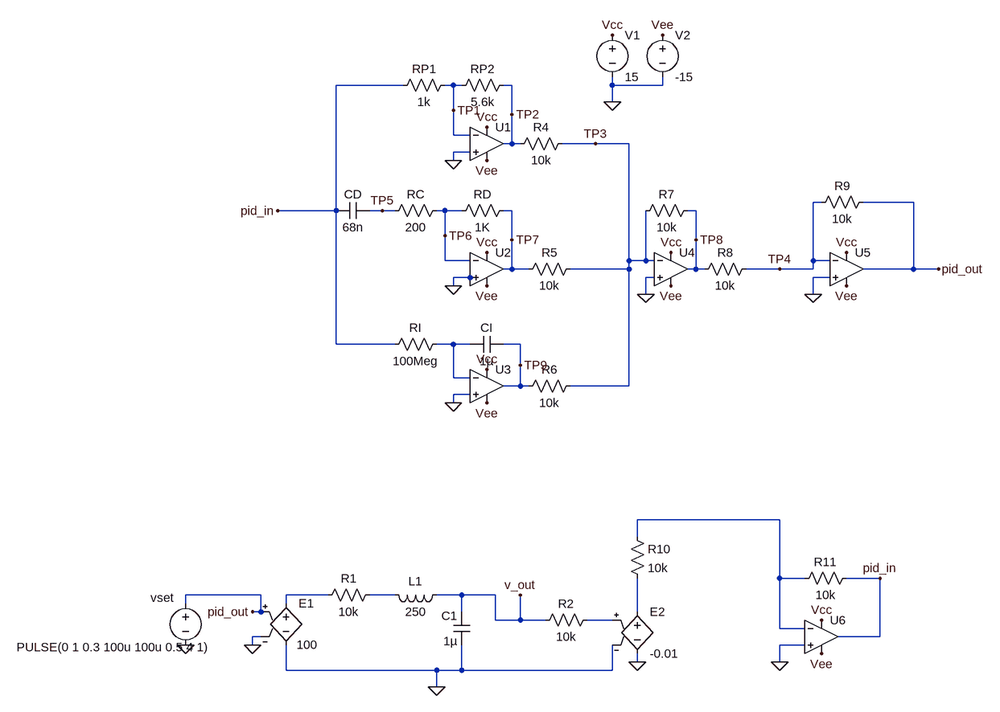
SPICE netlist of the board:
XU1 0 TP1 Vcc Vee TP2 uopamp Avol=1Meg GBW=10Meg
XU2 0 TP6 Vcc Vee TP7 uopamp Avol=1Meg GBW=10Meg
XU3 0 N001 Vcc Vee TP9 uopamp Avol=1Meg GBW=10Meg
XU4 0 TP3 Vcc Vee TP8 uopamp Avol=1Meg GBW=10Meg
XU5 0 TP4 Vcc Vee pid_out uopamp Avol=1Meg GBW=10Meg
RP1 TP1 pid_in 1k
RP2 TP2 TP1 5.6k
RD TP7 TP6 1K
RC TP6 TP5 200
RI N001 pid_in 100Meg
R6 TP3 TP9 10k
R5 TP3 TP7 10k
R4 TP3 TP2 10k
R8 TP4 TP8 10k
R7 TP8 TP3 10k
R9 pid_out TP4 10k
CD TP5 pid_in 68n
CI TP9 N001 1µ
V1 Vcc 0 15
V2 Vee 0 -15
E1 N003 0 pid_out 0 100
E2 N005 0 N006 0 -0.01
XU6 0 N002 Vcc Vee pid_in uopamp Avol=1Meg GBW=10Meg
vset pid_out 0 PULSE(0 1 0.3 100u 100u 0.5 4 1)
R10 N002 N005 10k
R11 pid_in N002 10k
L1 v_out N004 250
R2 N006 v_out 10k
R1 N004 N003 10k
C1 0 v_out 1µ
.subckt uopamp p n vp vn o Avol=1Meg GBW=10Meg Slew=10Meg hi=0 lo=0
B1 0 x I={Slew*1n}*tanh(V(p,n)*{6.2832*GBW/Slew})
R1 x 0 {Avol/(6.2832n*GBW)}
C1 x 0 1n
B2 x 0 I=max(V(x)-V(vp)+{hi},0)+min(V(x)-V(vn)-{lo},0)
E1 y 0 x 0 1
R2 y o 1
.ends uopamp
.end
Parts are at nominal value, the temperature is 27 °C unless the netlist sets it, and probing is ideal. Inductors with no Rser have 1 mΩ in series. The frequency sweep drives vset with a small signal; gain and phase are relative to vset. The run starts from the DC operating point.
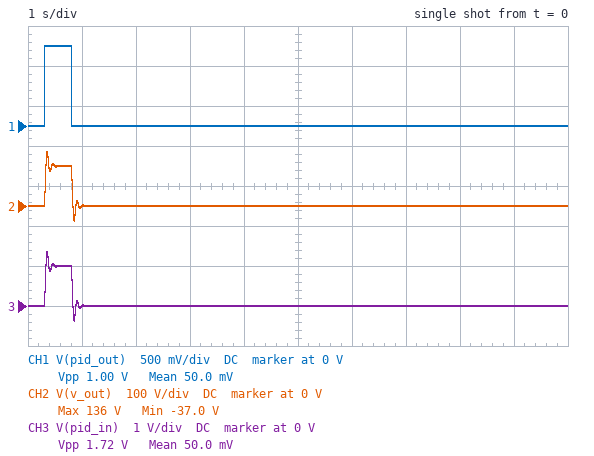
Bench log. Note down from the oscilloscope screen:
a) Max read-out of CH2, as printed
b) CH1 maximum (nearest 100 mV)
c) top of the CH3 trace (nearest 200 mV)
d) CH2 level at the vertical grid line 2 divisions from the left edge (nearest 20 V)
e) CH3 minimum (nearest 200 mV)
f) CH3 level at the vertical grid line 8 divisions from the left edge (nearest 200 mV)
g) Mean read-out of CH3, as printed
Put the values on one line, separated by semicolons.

136 V; 1.0 V; 1.4 V; 0 V; -400 mV; 0 V; 50.0 mV
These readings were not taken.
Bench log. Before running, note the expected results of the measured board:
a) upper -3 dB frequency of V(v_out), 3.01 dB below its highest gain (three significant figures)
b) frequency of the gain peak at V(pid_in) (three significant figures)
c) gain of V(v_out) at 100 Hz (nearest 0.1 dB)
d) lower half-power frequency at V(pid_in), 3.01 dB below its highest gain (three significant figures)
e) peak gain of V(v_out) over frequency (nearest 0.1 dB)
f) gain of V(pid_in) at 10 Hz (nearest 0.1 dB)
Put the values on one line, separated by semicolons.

11.9 Hz; 9.00 Hz; 0.2 dB; 4.50 Hz; 44.4 dB; 4.0 dB
